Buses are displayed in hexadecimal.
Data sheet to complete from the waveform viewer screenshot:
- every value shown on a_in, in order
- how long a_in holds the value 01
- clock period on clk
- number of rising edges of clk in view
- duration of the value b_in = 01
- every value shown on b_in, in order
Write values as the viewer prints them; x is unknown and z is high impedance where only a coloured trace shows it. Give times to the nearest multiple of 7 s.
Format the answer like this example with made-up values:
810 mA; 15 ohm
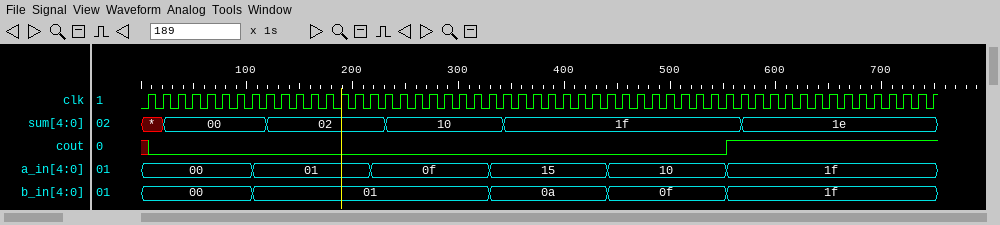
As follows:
00, 01, 0f, 15, 10, 1f; 112 s; 14 s; 54; 224 s; 00, 01, 0a, 0f, 1f
